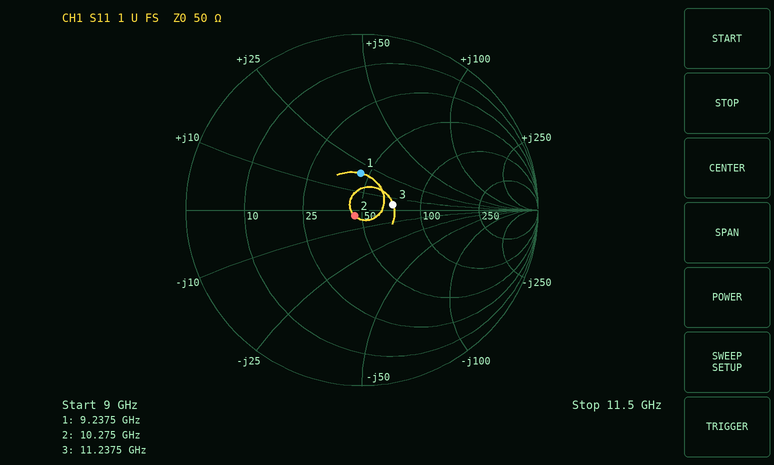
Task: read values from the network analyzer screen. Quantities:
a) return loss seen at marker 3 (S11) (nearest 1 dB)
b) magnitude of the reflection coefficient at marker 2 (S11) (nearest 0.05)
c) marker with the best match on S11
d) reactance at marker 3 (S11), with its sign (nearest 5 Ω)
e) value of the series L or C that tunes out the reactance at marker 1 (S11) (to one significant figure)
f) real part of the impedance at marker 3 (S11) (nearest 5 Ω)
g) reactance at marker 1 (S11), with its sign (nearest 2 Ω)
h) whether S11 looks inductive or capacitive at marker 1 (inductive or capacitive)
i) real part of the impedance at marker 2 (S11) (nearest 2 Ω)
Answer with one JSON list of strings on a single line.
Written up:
["15 dB", "0.05", "marker 2", "+5 Ω", "900 fF", "70 Ω", "+20 Ω", "inductive", "46 Ω"]
